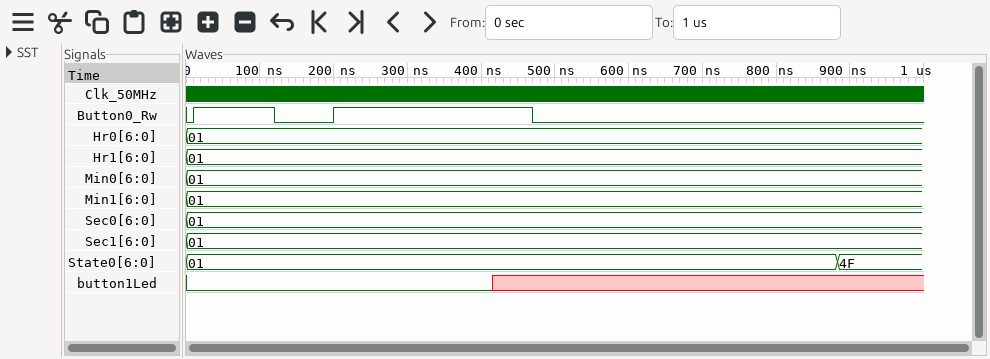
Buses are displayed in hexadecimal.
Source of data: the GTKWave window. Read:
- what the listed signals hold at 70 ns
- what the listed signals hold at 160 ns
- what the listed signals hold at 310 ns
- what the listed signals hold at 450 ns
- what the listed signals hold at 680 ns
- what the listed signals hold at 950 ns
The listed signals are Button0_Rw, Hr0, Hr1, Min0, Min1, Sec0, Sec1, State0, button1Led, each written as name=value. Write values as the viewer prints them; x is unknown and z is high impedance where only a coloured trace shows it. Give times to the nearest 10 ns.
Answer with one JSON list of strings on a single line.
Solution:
["Button0_Rw=1, Hr0=01, Hr1=01, Min0=01, Min1=01, Sec0=01, Sec1=01, State0=01, button1Led=0", "Button0_Rw=0, Hr0=01, Hr1=01, Min0=01, Min1=01, Sec0=01, Sec1=01, State0=01, button1Led=0", "Button0_Rw=1, Hr0=01, Hr1=01, Min0=01, Min1=01, Sec0=01, Sec1=01, State0=01, button1Led=0", "Button0_Rw=1, Hr0=01, Hr1=01, Min0=01, Min1=01, Sec0=01, Sec1=01, State0=01, button1Led=x", "Button0_Rw=0, Hr0=01, Hr1=01, Min0=01, Min1=01, Sec0=01, Sec1=01, State0=01, button1Led=x", "Button0_Rw=0, Hr0=01, Hr1=01, Min0=01, Min1=01, Sec0=01, Sec1=01, State0=4F, button1Led=x"]
